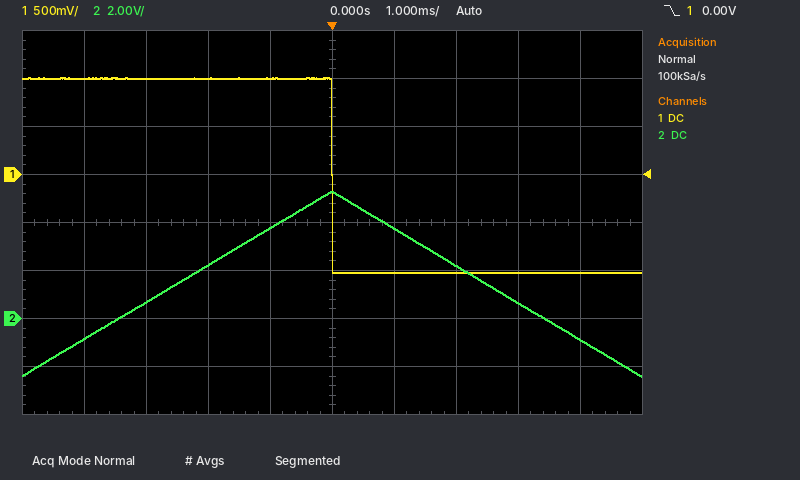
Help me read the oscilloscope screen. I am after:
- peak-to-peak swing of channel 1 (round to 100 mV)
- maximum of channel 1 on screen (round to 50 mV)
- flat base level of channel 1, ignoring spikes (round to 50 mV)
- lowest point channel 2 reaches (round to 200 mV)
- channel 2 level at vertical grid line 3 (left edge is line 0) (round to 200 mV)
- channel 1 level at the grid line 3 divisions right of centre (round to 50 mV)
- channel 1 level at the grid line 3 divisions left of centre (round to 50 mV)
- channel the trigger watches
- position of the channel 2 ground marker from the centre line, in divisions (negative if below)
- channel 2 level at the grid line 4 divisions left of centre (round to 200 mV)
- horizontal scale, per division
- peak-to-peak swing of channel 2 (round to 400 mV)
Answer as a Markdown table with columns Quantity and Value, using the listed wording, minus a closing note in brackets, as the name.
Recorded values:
| Quantity | Value |
|---|---|
| peak-to-peak swing of channel 1 | 2.00 V |
| maximum of channel 1 on screen | 1.00 V |
| flat base level of channel 1, ignoring spikes | -1.00 V |
| lowest point channel 2 reaches | -2.4 V |
| channel 2 level at vertical grid line 3 (left edge is line 0) | 2.2 V |
| channel 1 level at the grid line 3 divisions right of centre | -1.00 V |
| channel 1 level at the grid line 3 divisions left of centre | 1.00 V |
| channel the trigger watches | channel 1 |
| position of the channel 2 ground marker from the centre line, in divisions | -2.0 div |
| channel 2 level at the grid line 4 divisions left of centre | -800 mV |
| horizontal scale, per division | 1 ms |
| peak-to-peak swing of channel 2 | 7.6 V |
